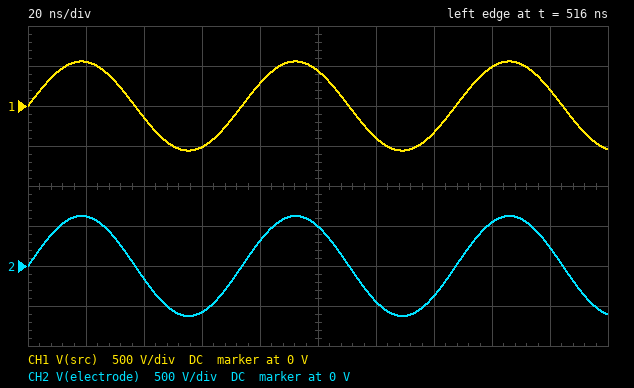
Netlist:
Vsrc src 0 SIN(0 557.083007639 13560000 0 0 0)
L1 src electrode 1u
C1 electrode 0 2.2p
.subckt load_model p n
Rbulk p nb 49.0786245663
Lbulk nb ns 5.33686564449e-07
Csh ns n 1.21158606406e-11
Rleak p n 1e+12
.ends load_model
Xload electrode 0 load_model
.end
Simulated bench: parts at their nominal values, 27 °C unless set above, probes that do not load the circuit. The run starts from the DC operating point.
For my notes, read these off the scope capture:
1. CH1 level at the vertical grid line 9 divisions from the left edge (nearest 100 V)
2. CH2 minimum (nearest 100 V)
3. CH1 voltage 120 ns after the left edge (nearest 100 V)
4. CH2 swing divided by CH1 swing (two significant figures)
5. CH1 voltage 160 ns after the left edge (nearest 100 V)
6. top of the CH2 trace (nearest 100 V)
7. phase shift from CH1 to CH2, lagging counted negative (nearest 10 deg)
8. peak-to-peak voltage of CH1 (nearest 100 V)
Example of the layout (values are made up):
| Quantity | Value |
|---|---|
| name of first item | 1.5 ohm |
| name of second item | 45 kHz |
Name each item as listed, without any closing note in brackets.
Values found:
| Quantity | Value |
|---|---|
| CH1 level at the vertical grid line 9 divisions from the left edge | 200 V |
| CH2 minimum | -600 V |
| CH1 voltage 120 ns after the left edge | -400 V |
| CH2 swing divided by CH1 swing | 1.1 |
| CH1 voltage 160 ns after the left edge | 500 V |
| top of the CH2 trace | 600 V |
| phase shift from CH1 to CH2, lagging counted negative | 0 deg |
| peak-to-peak voltage of CH1 | 1.1 kV |
